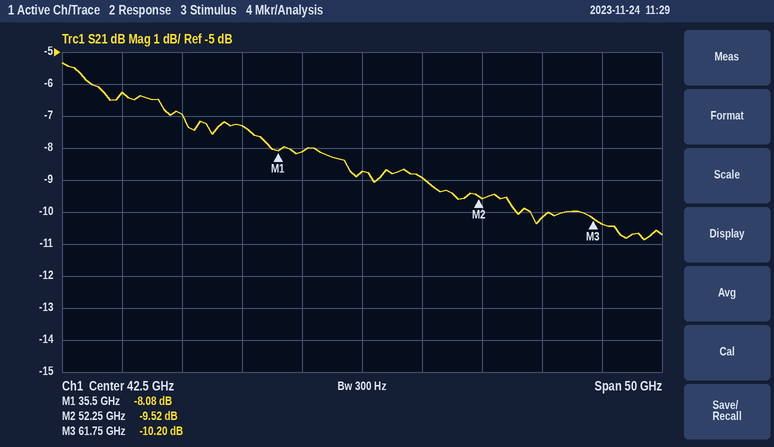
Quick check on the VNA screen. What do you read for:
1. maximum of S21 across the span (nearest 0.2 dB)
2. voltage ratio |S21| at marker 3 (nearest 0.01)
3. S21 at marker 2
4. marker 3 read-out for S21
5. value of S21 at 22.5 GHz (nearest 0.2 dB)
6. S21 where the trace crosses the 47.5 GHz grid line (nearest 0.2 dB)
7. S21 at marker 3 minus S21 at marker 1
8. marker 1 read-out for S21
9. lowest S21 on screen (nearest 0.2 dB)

-5.4 dB
0.31
-9.52 dB
-10.20 dB
-6.2 dB
-9.0 dB
-2.12 dB
-8.08 dB
-10.8 dB
